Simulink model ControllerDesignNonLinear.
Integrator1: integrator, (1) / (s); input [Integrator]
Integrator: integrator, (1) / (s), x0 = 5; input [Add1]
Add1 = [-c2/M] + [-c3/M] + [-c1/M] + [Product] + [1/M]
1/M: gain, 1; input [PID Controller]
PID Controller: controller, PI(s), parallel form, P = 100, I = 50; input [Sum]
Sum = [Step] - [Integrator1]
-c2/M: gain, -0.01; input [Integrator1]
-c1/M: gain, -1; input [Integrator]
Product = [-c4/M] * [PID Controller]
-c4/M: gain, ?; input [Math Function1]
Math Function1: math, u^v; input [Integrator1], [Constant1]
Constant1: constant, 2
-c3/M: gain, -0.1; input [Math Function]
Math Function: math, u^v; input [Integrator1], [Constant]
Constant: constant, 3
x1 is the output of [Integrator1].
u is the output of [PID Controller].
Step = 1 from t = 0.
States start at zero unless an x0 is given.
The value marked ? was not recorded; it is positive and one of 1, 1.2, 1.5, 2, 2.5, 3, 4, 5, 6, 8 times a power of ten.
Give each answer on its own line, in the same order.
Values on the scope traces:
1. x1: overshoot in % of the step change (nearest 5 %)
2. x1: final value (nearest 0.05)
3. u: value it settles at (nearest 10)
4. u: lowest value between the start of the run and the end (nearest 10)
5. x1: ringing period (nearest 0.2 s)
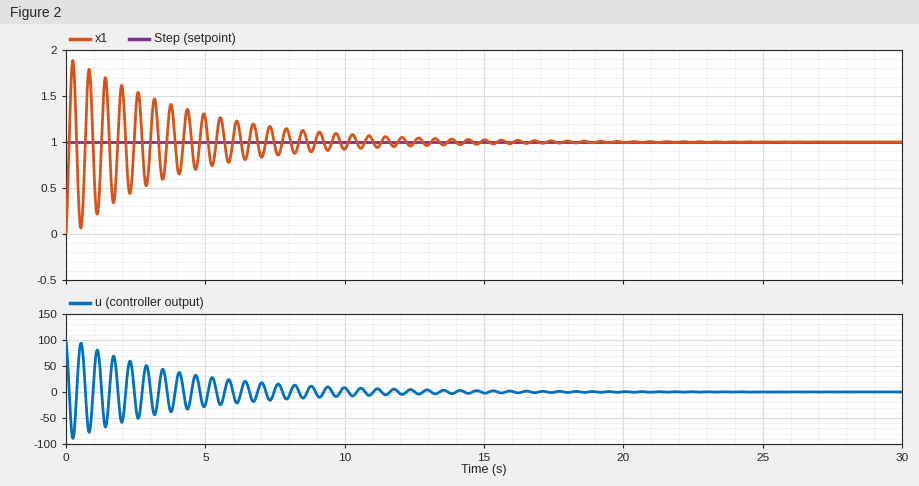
90 %
1.00
0
-90
0.6 s
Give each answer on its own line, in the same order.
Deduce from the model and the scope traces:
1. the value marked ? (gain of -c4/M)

0.12
